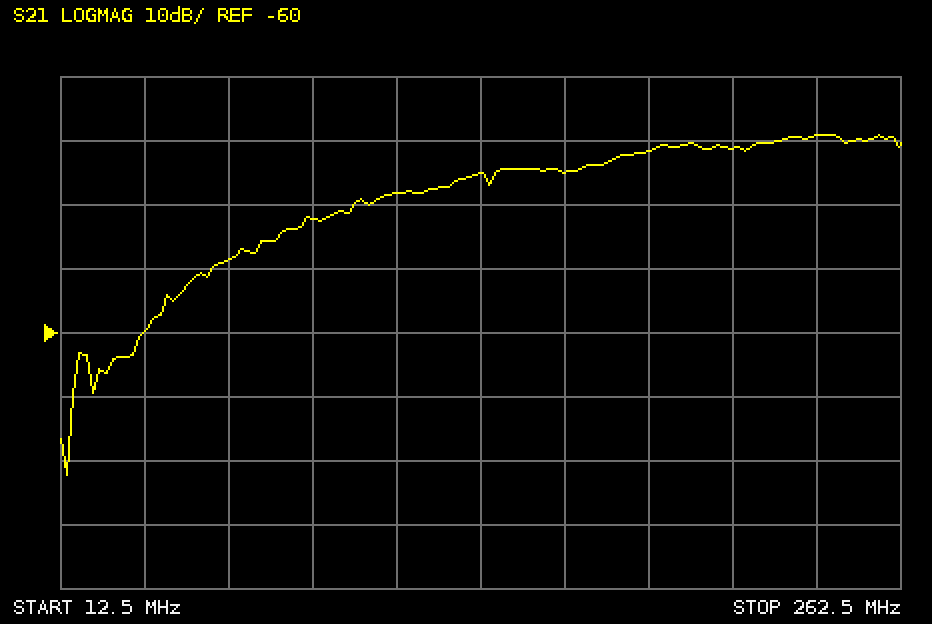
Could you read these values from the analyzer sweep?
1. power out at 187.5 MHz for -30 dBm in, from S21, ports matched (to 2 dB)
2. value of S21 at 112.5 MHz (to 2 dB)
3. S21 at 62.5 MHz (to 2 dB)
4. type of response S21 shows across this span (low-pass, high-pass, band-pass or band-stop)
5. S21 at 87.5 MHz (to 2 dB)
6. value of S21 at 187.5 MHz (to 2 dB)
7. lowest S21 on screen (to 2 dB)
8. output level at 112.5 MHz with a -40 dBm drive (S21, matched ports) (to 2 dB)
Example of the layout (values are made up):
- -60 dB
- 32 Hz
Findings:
- -62 dBm
- -38 dB
- -48 dB
- high-pass
- -42 dB
- -32 dB
- -82 dB
- -78 dBm
